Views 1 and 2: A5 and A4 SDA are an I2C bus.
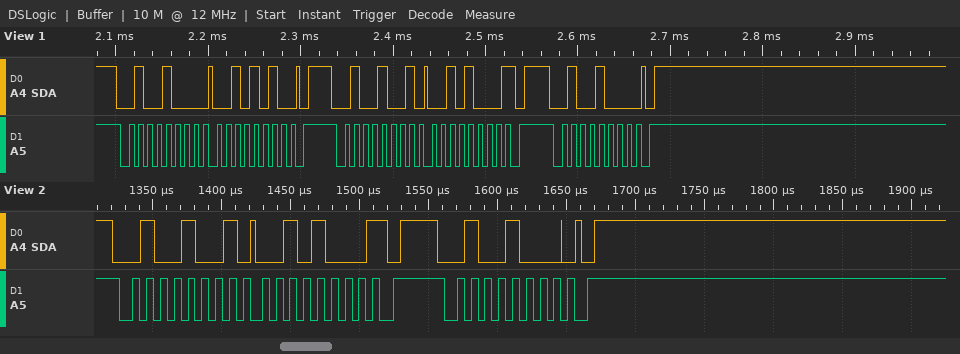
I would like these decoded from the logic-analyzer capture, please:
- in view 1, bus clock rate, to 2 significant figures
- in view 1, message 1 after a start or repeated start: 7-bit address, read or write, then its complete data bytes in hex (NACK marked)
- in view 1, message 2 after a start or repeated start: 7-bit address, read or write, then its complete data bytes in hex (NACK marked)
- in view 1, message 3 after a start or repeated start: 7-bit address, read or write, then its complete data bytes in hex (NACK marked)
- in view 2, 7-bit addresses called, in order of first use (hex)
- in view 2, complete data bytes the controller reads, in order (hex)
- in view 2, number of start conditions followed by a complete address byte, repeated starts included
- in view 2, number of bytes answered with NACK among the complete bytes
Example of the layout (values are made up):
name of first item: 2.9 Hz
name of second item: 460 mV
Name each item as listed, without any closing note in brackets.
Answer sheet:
in view 1, bus clock rate, to 2 significant figures: 100 kHz
in view 1, message 1 after a start or repeated start: 7-bit address, read or write, then its complete data bytes in hex: 0x24 write: 2A
in view 1, message 2 after a start or repeated start: 7-bit address, read or write, then its complete data bytes in hex: 0x24 read: 28 NACK
in view 1, message 3 after a start or repeated start: 7-bit address, read or write, then its complete data bytes in hex: 0x24 write
in view 2, 7-bit addresses called, in order of first use: 0x24
in view 2, complete data bytes the controller reads, in order: 28
in view 2, number of start conditions followed by a complete address byte, repeated starts included: 2
in view 2, number of bytes answered with NACK among the complete bytes: 1
